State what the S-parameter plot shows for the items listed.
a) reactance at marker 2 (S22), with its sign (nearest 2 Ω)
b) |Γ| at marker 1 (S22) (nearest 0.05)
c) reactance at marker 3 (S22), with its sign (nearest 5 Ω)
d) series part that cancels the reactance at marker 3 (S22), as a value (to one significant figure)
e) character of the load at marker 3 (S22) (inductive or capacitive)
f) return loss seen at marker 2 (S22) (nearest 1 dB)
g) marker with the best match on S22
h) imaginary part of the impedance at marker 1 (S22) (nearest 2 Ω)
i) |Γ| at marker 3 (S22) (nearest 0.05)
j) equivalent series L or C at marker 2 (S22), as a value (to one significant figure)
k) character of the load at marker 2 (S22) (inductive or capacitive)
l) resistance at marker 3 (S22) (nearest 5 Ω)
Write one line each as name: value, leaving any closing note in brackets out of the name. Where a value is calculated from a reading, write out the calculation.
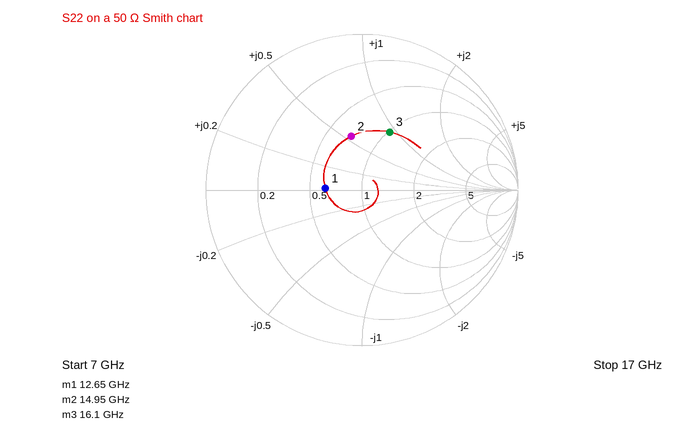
reactance at marker 2 (S22), with its sign: +28 Ω
|Γ| at marker 1 (S22): 0.25
reactance at marker 3 (S22), with its sign: +45 Ω
series part that cancels the reactance at marker 3 (S22), as a value: C = 1/(2π × 16.1 GHz × 45 Ω) ≈ 220 fF, so 200 fF to one significant figure
character of the load at marker 3 (S22): inductive
return loss seen at marker 2 (S22): 9 dB
marker with the best match on S22: marker 1
imaginary part of the impedance at marker 1 (S22): 0 Ω
|Γ| at marker 3 (S22): 0.40
equivalent series L or C at marker 2 (S22), as a value: L = 28 Ω/(2π × 14.95 GHz) ≈ 298 pH, so 300 pH to one significant figure
character of the load at marker 2 (S22): inductive
resistance at marker 3 (S22): 50 Ω
